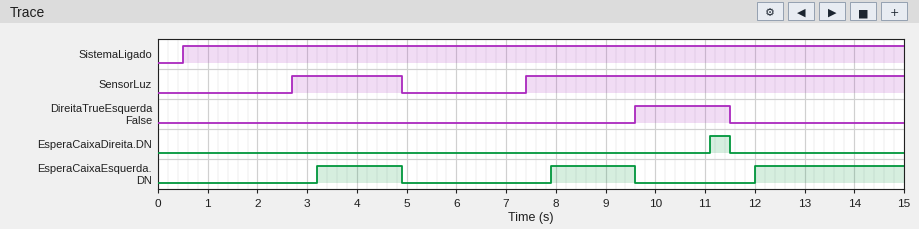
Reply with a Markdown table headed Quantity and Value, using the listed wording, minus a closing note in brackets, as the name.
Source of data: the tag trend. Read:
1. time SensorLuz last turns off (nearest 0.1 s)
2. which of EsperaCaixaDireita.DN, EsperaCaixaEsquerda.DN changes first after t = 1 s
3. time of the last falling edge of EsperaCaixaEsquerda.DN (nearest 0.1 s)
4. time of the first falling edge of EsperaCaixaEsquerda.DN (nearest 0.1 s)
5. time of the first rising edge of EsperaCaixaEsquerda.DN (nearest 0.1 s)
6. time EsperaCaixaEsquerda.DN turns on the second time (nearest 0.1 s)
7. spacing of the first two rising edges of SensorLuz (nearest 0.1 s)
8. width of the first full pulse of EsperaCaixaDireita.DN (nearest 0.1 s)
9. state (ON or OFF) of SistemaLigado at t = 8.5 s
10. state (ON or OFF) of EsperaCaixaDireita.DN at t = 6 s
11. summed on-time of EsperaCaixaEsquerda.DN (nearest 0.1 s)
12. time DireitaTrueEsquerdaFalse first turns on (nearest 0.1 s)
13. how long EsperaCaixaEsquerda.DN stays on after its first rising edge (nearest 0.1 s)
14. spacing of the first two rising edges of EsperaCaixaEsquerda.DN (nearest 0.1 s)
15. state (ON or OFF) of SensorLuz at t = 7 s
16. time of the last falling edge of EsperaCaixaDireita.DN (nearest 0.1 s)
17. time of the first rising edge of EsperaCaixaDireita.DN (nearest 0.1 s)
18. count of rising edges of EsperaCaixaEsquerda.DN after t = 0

| Quantity | Value |
|---|---|
| time SensorLuz last turns off | 4.9 s |
| which of EsperaCaixaDireita.DN, EsperaCaixaEsquerda.DN changes first after t = 1 s | EsperaCaixaEsquerda.DN |
| time of the last falling edge of EsperaCaixaEsquerda.DN | 9.6 s |
| time of the first falling edge of EsperaCaixaEsquerda.DN | 4.9 s |
| time of the first rising edge of EsperaCaixaEsquerda.DN | 3.2 s |
| time EsperaCaixaEsquerda.DN turns on the second time | 7.9 s |
| spacing of the first two rising edges of SensorLuz | 4.7 s |
| width of the first full pulse of EsperaCaixaDireita.DN | 0.4 s |
| state (ON or OFF) of SistemaLigado at t = 8.5 s | ON |
| state (ON or OFF) of EsperaCaixaDireita.DN at t = 6 s | OFF |
| summed on-time of EsperaCaixaEsquerda.DN | 6.4 s |
| time DireitaTrueEsquerdaFalse first turns on | 9.6 s |
| how long EsperaCaixaEsquerda.DN stays on after its first rising edge | 1.7 s |
| spacing of the first two rising edges of EsperaCaixaEsquerda.DN | 4.7 s |
| state (ON or OFF) of SensorLuz at t = 7 s | OFF |
| time of the last falling edge of EsperaCaixaDireita.DN | 11.5 s |
| time of the first rising edge of EsperaCaixaDireita.DN | 11.1 s |
| count of rising edges of EsperaCaixaEsquerda.DN after t = 0 | 3 |
